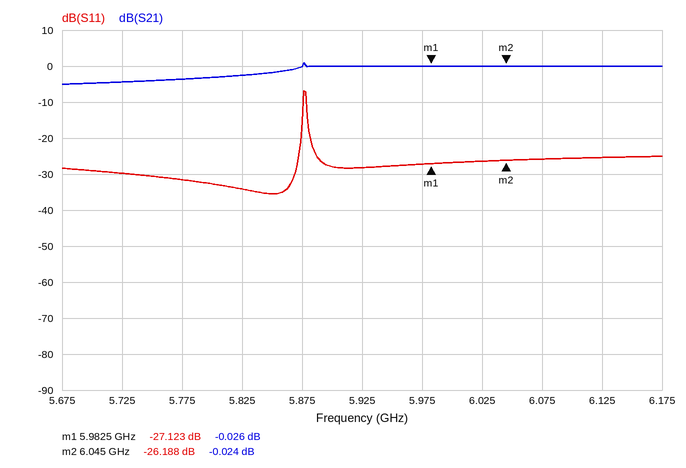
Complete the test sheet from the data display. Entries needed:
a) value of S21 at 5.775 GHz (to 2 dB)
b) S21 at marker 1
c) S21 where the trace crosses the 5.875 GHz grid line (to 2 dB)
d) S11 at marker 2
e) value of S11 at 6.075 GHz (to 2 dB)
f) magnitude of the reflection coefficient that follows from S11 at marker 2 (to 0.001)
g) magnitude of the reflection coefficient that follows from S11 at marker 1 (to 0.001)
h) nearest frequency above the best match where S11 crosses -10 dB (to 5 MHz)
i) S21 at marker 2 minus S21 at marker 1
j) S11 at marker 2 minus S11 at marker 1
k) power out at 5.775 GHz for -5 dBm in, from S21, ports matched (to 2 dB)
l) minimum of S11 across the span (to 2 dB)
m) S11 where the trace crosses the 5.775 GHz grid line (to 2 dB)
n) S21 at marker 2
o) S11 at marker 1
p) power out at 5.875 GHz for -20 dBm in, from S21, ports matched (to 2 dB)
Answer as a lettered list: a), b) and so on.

a) -4 dB
b) -0.026 dB
c) 0 dB
d) -26.188 dB
e) -26 dB
f) 0.049
g) 0.044
h) 5.875 GHz
i) 0.002 dB
j) 0.935 dB
k) -8 dBm
l) -36 dB
m) -32 dB
n) -0.024 dB
o) -27.123 dB
p) -20 dBm
